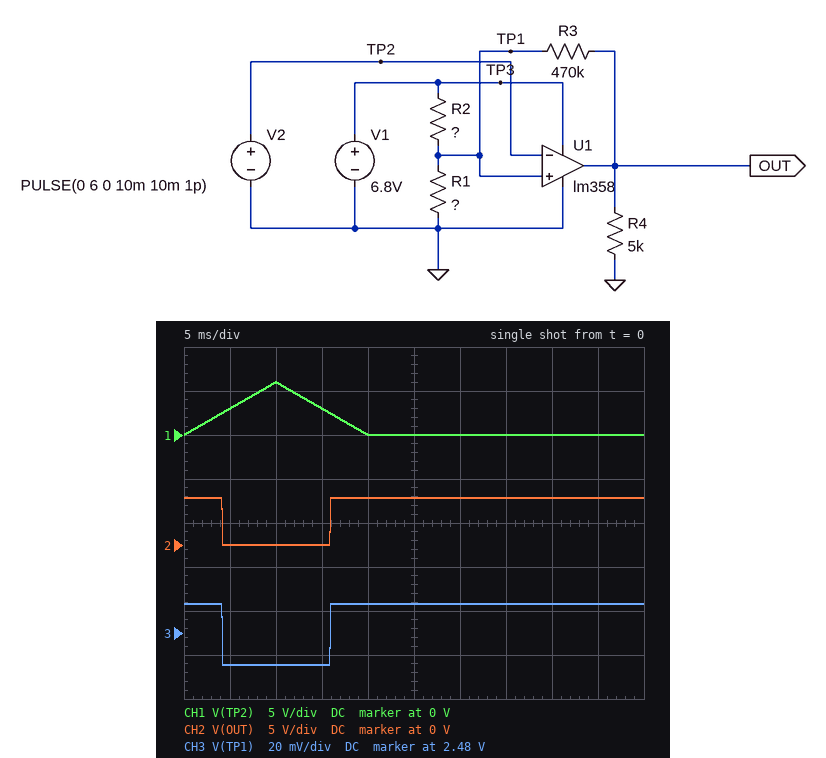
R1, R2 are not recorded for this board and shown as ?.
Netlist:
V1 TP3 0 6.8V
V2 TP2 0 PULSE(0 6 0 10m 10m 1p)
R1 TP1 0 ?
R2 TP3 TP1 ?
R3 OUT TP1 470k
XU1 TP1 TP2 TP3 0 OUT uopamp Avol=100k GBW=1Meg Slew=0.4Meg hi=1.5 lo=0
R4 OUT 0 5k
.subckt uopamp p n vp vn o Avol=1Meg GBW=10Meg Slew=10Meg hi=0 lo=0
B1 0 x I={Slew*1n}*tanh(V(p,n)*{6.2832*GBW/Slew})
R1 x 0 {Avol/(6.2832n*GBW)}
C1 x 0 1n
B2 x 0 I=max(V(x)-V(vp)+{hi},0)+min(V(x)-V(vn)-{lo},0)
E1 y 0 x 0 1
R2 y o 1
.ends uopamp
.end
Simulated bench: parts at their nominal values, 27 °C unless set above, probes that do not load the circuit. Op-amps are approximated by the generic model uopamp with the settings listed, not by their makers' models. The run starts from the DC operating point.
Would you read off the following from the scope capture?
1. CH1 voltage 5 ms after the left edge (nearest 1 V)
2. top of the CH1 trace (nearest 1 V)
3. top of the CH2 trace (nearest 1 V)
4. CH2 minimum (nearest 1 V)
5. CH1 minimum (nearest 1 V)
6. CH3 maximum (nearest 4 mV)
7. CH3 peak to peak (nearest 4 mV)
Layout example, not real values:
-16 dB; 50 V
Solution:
3 V; 6 V; 5 V; 0 V; 0 V; 2.492 V; 28 mV
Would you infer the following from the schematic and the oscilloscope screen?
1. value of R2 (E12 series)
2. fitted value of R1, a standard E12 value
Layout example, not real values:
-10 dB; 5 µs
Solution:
6.8 kΩ; 3.9 kΩ
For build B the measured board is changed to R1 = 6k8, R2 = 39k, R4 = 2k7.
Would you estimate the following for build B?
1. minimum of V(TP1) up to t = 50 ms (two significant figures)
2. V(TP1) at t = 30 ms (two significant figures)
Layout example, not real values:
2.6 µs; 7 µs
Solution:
1.0 V; 1.1 V
